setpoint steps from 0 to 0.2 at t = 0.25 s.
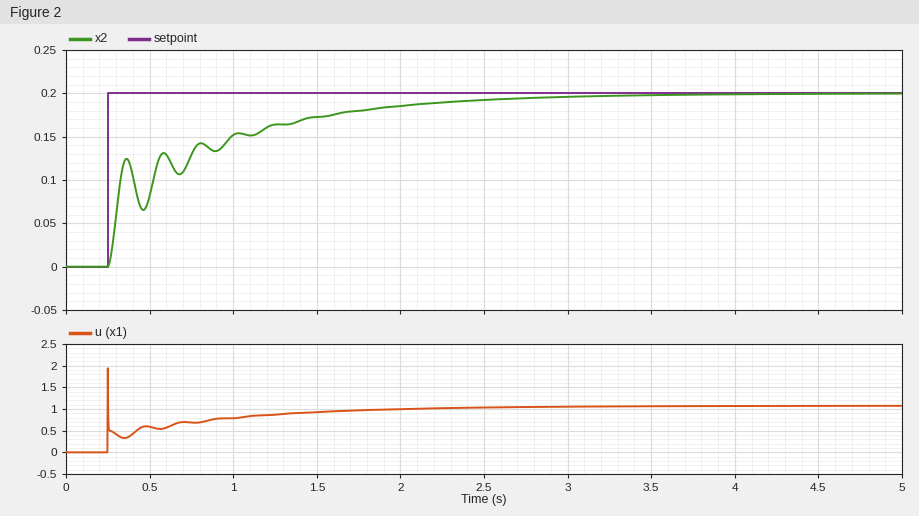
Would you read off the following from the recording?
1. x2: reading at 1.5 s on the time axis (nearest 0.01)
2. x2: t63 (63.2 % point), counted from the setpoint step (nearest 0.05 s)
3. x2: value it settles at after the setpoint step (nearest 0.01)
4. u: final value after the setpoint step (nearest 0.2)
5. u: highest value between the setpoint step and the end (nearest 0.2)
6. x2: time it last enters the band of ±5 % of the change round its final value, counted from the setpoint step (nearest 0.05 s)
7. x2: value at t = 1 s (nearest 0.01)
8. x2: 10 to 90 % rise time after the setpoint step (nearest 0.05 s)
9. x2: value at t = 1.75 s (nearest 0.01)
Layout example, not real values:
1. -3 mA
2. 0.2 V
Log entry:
1. 0.17
2. 0.30 s
3. 0.20
4. 1.0
5. 2.0
6. 2.05 s
7. 0.15
8. 1.50 s
9. 0.18
